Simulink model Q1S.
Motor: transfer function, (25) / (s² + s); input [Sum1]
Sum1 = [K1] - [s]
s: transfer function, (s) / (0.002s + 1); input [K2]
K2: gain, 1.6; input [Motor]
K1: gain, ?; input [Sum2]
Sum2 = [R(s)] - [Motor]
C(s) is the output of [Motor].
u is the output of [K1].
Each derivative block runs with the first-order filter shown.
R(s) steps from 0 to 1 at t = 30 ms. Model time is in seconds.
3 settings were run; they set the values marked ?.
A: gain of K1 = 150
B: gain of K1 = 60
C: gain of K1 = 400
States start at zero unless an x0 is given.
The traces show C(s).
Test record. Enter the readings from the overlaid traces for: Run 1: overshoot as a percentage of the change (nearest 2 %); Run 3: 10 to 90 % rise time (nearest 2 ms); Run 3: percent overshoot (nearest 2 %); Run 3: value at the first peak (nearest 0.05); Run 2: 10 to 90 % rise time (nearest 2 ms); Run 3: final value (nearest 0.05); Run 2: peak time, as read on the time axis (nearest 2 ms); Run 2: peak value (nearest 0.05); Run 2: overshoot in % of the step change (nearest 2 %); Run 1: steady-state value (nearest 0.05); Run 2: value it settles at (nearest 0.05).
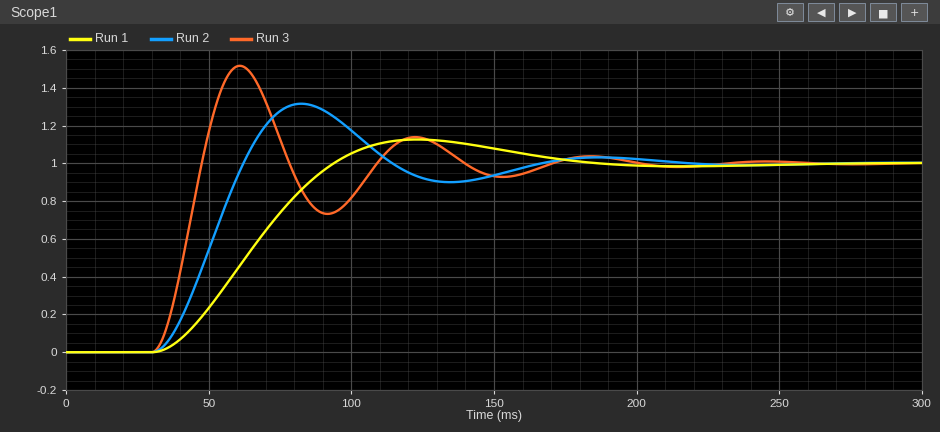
12 %
12 ms
52 %
1.50
22 ms
1.00
82 ms
1.30
32 %
1.00
1.00
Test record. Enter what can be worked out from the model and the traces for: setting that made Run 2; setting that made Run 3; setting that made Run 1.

A
C
B
